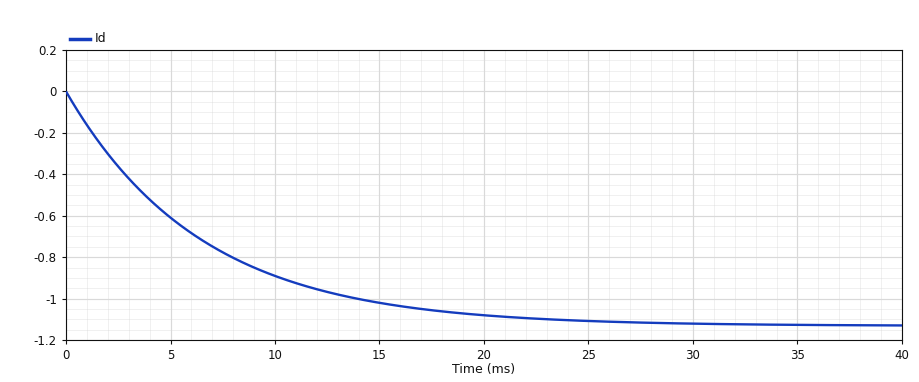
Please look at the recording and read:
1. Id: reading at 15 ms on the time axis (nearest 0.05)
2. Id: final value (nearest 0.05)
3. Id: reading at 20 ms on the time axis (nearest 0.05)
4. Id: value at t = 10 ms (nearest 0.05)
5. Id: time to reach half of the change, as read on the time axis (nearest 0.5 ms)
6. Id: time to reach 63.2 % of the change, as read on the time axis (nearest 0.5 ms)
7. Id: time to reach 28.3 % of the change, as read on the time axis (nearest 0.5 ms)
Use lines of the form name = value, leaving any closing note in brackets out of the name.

Id: reading at 15 ms on the time axis = -1.00
Id: final value = -1.15
Id: reading at 20 ms on the time axis = -1.10
Id: value at t = 10 ms = -0.90
Id: time to reach half of the change, as read on the time axis = 4.5 ms
Id: time to reach 63.2 % of the change, as read on the time axis = 6.5 ms
Id: time to reach 28.3 % of the change, as read on the time axis = 2.0 ms
